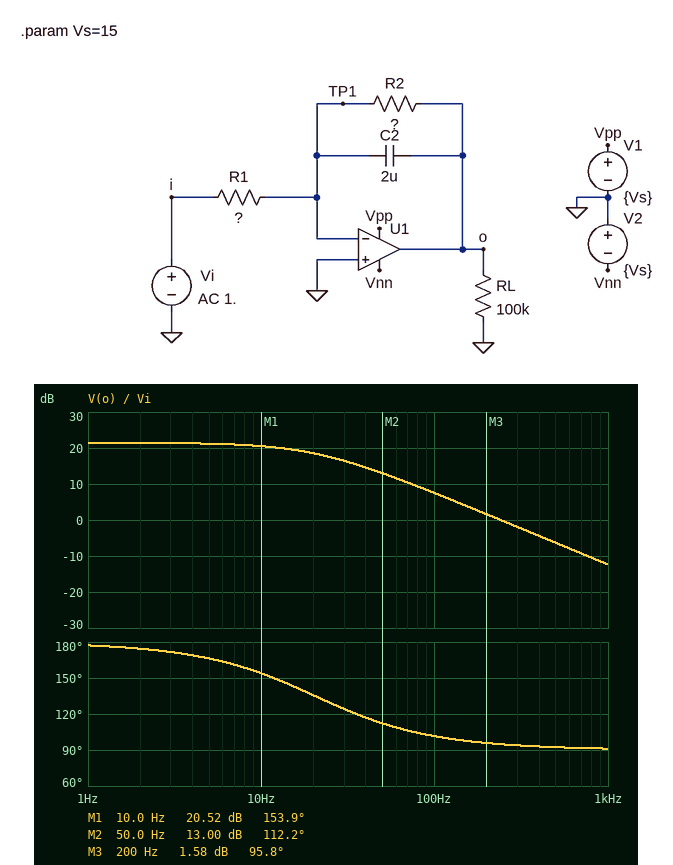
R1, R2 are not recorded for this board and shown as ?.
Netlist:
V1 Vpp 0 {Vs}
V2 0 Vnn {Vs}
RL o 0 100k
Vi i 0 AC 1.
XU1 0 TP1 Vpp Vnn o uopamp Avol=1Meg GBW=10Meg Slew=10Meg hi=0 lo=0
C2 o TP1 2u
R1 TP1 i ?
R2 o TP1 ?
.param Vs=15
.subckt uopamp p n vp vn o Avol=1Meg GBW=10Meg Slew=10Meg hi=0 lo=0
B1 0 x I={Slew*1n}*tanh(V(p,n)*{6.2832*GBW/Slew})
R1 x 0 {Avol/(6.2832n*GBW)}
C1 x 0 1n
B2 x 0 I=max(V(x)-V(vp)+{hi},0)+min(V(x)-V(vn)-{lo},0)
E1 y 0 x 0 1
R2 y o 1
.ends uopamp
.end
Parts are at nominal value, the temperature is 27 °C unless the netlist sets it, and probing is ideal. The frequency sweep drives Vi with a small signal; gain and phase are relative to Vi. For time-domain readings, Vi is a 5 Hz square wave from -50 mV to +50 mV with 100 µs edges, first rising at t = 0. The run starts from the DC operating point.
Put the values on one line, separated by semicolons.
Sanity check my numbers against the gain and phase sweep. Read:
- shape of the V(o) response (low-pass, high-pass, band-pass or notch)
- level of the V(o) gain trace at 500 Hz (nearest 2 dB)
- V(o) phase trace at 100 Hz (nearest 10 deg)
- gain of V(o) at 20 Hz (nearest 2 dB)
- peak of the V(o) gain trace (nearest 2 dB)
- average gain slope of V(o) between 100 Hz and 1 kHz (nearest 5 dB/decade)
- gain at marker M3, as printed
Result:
low-pass; -6 dB; 100 deg; 18 dB; 22 dB; -20 dB/decade; 1.58 dB
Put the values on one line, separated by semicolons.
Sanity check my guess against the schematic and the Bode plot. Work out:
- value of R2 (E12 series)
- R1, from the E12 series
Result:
3.9 kΩ; 330 Ω
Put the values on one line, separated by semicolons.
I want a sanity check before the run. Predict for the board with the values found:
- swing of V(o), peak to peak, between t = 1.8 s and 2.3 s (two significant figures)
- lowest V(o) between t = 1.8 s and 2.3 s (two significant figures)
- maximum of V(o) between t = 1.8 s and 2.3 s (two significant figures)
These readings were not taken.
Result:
1.2 V; -590 mV; 590 mV
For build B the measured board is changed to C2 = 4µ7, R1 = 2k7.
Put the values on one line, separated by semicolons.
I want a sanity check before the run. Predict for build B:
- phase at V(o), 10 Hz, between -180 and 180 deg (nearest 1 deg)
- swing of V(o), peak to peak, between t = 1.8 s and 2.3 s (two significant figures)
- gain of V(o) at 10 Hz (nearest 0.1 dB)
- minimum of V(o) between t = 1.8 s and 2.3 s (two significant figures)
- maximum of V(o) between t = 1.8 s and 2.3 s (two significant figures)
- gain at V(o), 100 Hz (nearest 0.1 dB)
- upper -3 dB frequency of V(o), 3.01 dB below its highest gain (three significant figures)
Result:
131 deg; 140 mV; -0.5 dB; -72 mV; 72 mV; -18.1 dB; 8.68 Hz
